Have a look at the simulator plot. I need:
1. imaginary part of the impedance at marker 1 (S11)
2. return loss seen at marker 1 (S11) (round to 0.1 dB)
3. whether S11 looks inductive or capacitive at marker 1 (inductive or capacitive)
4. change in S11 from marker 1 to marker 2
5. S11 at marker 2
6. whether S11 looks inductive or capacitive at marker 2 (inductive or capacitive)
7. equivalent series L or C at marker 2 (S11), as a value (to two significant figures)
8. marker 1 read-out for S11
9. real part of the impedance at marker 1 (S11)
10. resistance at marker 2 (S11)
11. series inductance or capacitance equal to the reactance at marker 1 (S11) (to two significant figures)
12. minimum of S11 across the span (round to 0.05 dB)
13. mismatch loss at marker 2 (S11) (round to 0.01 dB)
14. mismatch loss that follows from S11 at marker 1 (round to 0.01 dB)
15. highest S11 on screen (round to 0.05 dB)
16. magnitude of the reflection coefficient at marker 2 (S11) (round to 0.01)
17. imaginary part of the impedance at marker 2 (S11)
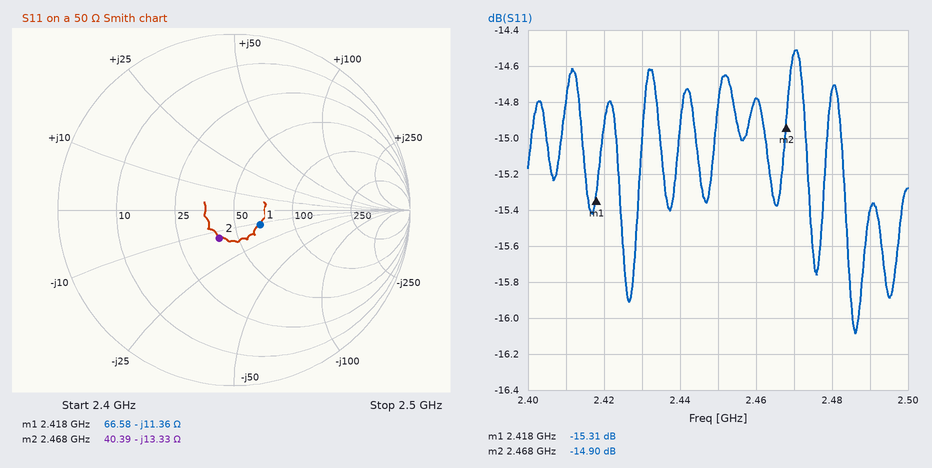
-11.36 Ω
15.3 dB
capacitive
0.41 dB
-14.90 dB
capacitive
4.8 pF
-15.31 dB
66.58 Ω
40.39 Ω
5.8 pF
-16.10 dB
0.14 dB
0.13 dB
-14.50 dB
0.18
-13.33 Ω
